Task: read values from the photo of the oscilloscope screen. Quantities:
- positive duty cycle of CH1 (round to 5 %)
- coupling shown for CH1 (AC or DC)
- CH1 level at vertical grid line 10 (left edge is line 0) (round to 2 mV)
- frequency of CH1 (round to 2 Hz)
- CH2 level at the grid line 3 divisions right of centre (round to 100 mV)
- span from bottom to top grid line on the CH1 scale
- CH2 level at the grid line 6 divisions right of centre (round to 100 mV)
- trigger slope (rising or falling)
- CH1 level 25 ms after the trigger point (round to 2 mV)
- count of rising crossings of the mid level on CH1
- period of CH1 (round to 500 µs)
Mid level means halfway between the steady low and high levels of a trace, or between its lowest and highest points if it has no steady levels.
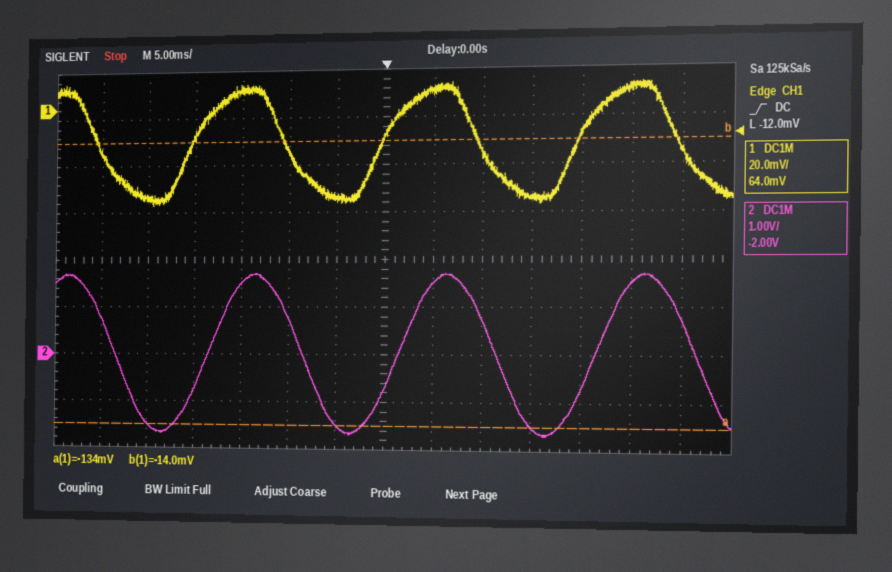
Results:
50 %
DC
-38 mV
50 Hz
-1.5 V
160 mV
700 mV
rising
8 mV
3
20.0 ms
